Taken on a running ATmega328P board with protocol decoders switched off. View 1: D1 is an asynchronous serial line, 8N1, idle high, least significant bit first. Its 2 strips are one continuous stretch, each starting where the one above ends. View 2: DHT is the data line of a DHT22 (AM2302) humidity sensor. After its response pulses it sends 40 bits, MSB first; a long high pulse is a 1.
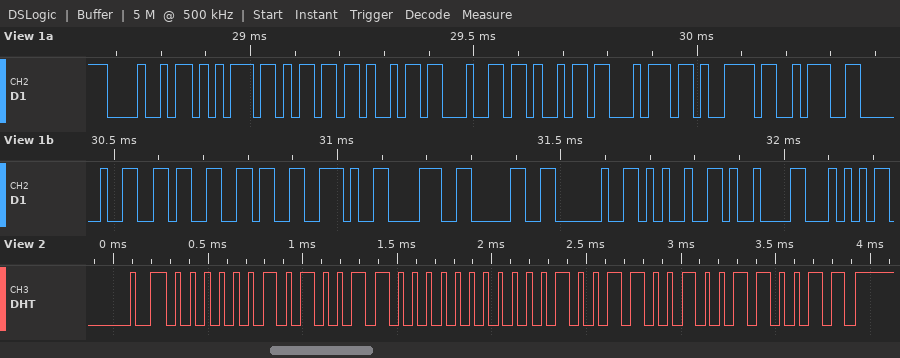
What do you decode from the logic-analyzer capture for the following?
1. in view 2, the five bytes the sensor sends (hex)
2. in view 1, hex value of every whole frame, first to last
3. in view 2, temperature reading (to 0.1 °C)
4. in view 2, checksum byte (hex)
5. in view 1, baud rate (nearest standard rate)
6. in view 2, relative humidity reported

02 98 00 99 33
48 75 6D 69 64 69 74 79 3A 20 36 36 2E 38 30 20 25 09 54
15.3 °C
0x33
57600 baud
66.4 %
